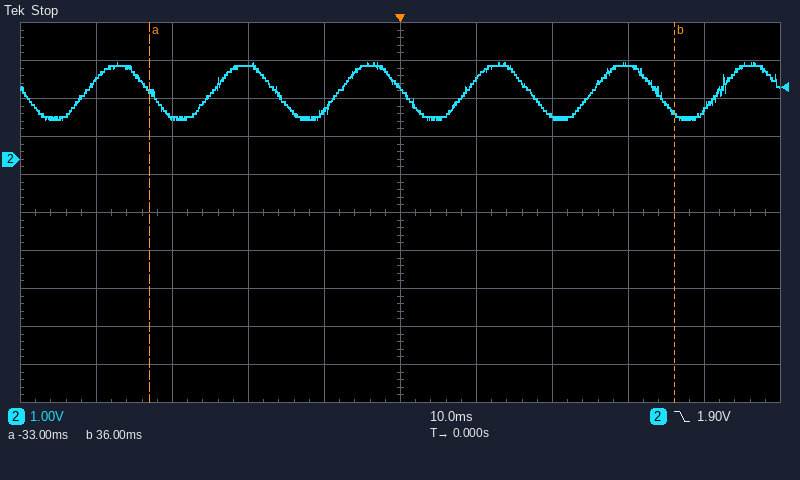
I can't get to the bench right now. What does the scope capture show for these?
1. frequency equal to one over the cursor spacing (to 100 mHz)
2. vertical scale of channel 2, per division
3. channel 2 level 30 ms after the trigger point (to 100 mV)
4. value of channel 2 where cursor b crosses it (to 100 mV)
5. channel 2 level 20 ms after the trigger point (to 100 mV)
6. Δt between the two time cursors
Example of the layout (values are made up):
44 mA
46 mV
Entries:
14.5 Hz
1 V
2.5 V
1.2 V
1.1 V
69 ms
